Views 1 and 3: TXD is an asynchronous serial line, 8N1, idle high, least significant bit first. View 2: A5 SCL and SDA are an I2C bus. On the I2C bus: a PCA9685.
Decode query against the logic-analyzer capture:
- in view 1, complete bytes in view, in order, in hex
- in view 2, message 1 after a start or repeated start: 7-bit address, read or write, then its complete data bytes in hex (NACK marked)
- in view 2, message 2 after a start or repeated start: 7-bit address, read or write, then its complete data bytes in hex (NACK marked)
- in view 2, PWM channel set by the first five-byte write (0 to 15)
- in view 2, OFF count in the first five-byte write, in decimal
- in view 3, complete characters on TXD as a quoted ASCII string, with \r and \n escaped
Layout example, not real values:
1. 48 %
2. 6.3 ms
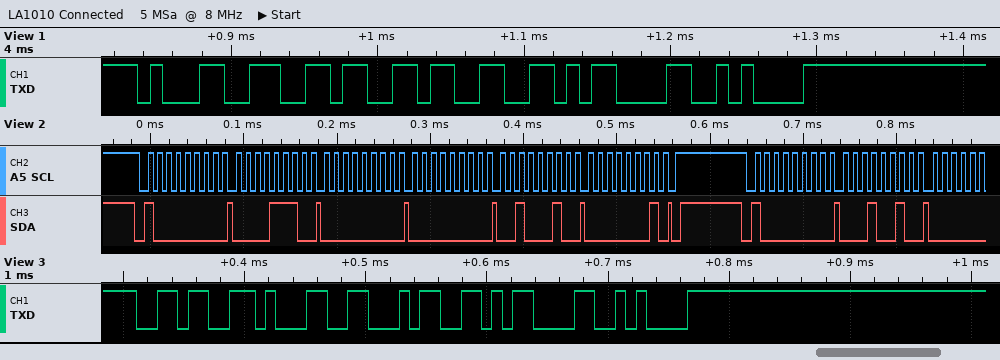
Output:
1. 31 36 33 0D 0A
2. 0x40 write: 0E 00 00 22 01
3. 0x40 write: 12
4. 2
5. 290
6. "614\r\n"
